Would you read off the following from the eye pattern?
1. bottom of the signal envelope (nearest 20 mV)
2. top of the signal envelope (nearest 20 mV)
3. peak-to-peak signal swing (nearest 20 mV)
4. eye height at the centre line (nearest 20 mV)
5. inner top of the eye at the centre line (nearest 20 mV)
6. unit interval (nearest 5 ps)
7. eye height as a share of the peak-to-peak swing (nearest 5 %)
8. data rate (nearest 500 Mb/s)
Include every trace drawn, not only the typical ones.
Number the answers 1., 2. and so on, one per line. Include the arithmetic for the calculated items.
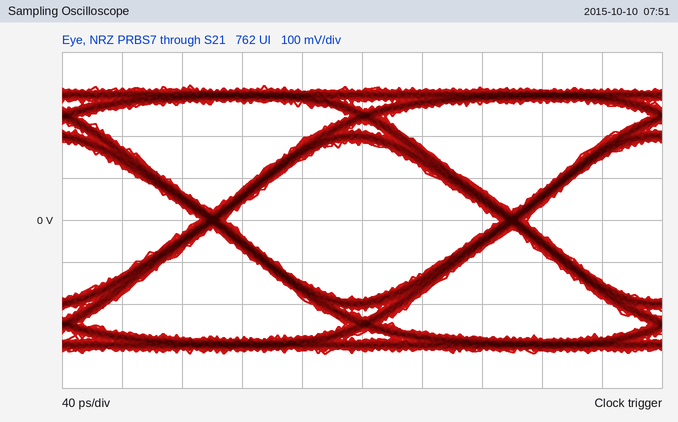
1. -320 mV
2. 320 mV
3. 640 mV
4. 380 mV
5. 180 mV
6. 200 ps
7. 380 mV / 640 mV ≈ 59.4 %, so 60 % to the nearest 5 %
8. 5.0 Gb/s
